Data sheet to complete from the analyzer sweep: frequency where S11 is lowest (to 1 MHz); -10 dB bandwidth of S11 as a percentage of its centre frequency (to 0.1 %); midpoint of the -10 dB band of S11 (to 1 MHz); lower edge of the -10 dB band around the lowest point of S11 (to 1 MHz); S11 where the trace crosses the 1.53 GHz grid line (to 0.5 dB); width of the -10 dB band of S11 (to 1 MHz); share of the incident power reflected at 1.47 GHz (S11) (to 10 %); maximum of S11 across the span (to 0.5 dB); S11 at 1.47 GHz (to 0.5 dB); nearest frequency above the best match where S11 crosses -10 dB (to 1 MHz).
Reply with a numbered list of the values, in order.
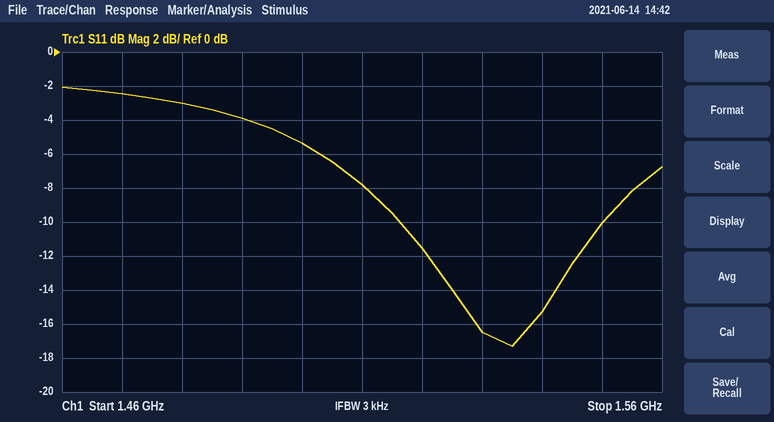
1. 1.535 GHz
2. 2.2 %
3. 1.533 GHz
4. 1.516 GHz
5. -16.5 dB
6. 34 MHz
7. 60 %
8. -2.0 dB
9. -2.5 dB
10. 1.550 GHz
